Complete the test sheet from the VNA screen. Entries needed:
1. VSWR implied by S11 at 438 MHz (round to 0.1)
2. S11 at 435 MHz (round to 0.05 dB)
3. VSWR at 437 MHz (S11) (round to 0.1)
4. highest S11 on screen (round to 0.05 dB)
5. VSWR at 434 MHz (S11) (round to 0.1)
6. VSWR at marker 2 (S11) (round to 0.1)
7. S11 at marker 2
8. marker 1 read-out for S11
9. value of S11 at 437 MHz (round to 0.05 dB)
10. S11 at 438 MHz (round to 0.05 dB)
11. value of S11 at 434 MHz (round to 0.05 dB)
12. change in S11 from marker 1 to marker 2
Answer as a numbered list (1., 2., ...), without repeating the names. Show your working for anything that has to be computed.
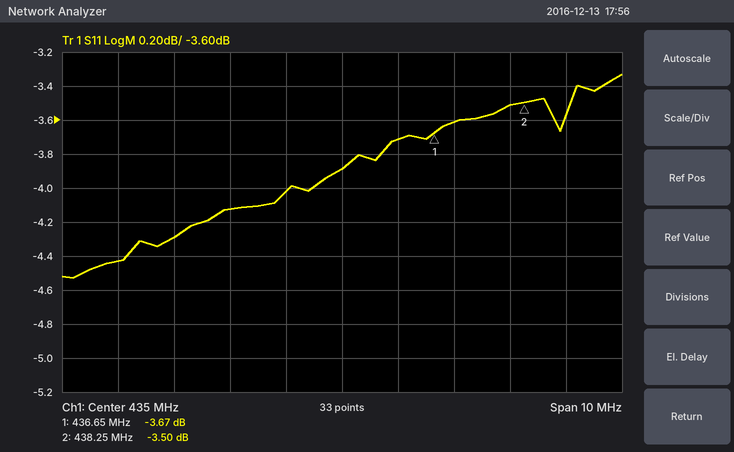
1. |Γ| = 10^(-3.5/20) = 0.6683; VSWR = (1 + 0.6683)/(1 − 0.6683) ≈ 5.0
2. -3.90 dB
3. |Γ| = 10^(-3.6/20) = 0.6607; VSWR = (1 + 0.6607)/(1 − 0.6607) ≈ 4.9
4. -3.35 dB
5. |Γ| = 10^(-4/20) = 0.6310; VSWR = (1 + 0.6310)/(1 − 0.6310) ≈ 4.4
6. (1 + 0.6683)/(1 − 0.6683) ≈ 5.0
7. -3.50 dB
8. -3.67 dB
9. -3.60 dB
10. -3.50 dB
11. -4.00 dB
12. -3.5 − (-3.67) = 0.17 dB
